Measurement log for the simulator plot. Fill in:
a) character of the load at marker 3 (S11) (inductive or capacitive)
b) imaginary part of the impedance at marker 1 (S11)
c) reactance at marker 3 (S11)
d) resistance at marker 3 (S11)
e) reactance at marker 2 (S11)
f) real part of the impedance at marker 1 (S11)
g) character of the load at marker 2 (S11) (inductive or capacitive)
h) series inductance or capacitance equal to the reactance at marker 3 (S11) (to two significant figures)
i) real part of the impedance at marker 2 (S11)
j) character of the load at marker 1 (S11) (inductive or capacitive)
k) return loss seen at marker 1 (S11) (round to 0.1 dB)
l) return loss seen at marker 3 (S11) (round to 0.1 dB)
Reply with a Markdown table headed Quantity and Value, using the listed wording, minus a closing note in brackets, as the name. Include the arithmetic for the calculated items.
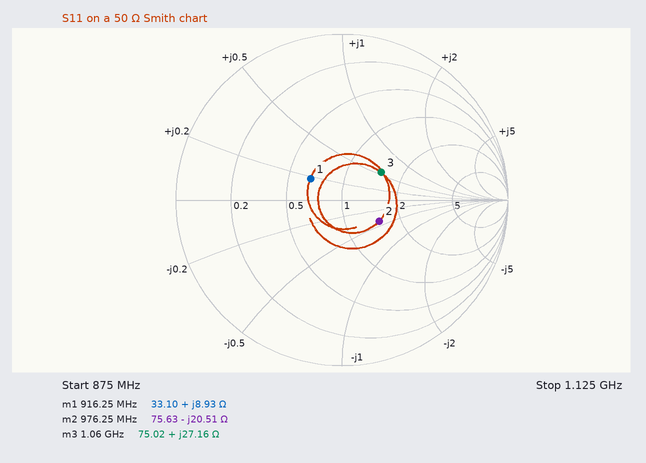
| Quantity | Value |
|---|---|
| character of the load at marker 3 (S11) | inductive |
| imaginary part of the impedance at marker 1 | +8.93 Ω |
| reactance at marker 3 | +27.16 Ω |
| resistance at marker 3 | 75.02 Ω |
| reactance at marker 2 | -20.51 Ω |
| real part of the impedance at marker 1 | 33.10 Ω |
| character of the load at marker 2 (S11) | capacitive |
| series inductance or capacitance equal to the reactance at marker 3 (S11) | L = 27.16 Ω/(2π × 1.06 GHz) ≈ 4.1 nH |
| real part of the impedance at marker 2 | 75.63 Ω |
| character of the load at marker 1 (S11) | inductive |
| return loss seen at marker 1 (S11) | 12.8 dB |
| return loss seen at marker 3 (S11) | 10.8 dB |
